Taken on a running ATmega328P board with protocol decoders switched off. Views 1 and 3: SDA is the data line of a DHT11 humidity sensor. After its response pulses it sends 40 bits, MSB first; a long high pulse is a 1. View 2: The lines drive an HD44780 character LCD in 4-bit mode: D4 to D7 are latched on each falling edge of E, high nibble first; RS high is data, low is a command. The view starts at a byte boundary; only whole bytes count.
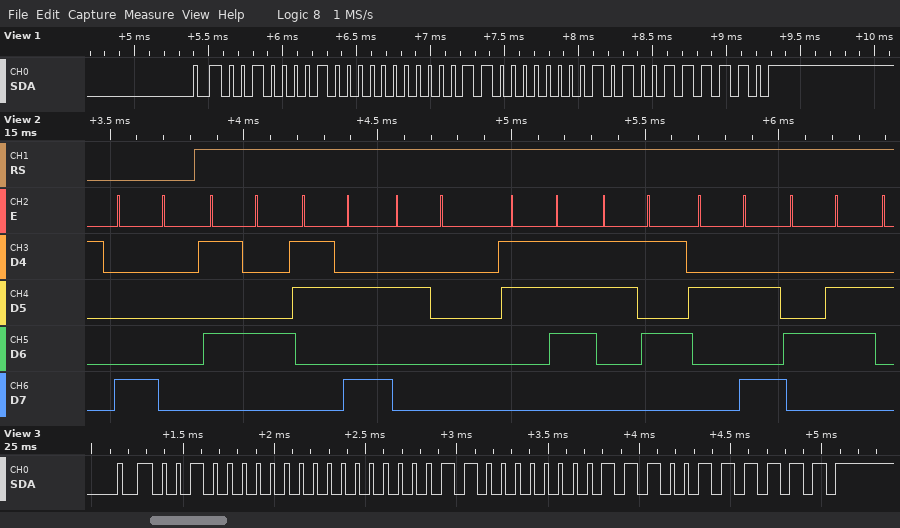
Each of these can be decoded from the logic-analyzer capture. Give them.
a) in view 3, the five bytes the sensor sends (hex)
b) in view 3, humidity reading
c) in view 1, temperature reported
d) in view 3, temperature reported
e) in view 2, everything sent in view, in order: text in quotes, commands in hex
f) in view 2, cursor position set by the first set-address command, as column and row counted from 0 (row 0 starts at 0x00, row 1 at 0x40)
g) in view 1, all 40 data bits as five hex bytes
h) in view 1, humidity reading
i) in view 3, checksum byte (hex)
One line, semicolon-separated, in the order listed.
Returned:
20 00 18 07 3F; 32 %; 24.5 °C; 24.7 °C; 0x80 "T: 75*F"; column 0, row 0; 21 00 18 05 3E; 33 %; 0x3F
